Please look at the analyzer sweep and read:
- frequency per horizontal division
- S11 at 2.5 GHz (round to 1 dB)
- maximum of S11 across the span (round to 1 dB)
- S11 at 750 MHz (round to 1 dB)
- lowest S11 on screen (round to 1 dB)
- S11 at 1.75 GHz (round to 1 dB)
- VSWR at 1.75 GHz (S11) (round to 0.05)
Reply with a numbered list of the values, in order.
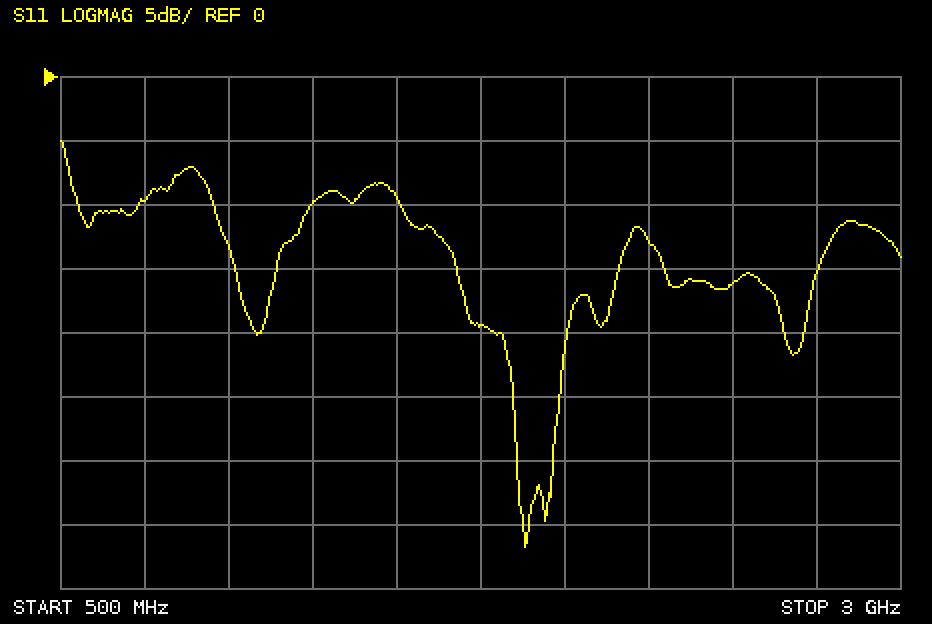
1. 250 MHz
2. -16 dB
3. -5 dB
4. -10 dB
5. -37 dB
6. -19 dB
7. 1.25
